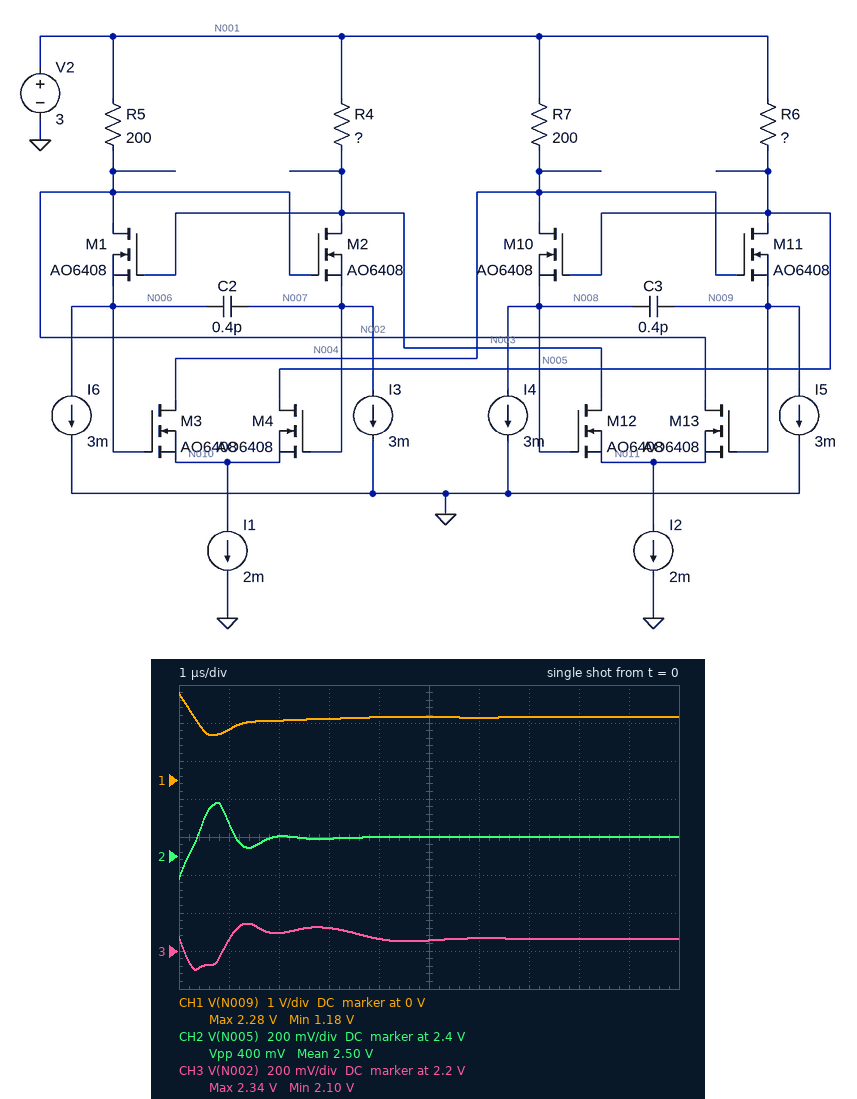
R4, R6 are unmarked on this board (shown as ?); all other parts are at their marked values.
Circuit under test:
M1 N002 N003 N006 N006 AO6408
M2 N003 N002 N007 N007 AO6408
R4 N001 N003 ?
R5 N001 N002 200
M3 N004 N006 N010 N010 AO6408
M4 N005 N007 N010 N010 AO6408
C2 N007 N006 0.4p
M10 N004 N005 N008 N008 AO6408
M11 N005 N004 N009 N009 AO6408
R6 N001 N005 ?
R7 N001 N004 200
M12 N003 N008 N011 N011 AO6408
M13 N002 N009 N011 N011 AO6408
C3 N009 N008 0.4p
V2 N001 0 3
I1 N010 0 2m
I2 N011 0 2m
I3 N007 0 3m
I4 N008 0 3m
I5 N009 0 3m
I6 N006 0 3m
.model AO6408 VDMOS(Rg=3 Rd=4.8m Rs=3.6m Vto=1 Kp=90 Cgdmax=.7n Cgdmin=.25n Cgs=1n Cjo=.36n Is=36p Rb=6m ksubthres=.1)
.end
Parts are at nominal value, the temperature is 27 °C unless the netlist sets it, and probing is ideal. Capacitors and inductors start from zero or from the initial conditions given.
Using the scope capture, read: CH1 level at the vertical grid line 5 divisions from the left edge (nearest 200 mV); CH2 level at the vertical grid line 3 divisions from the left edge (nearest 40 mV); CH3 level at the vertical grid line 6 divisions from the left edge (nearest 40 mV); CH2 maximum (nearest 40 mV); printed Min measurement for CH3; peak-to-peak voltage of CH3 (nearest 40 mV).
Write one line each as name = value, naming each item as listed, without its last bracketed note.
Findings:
CH1 level at the vertical grid line 5 divisions from the left edge = 1.6 V
CH2 level at the vertical grid line 3 divisions from the left edge = 2.48 V
CH3 level at the vertical grid line 6 divisions from the left edge = 2.28 V
CH2 maximum = 2.68 V
printed Min measurement for CH3 = 2.10 V
peak-to-peak voltage of CH3 = 240 mV
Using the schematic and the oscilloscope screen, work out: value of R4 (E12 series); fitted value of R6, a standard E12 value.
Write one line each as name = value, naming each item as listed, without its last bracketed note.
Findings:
value of R4 = 470 Ω
fitted value of R6, a standard E12 value = 100 Ω
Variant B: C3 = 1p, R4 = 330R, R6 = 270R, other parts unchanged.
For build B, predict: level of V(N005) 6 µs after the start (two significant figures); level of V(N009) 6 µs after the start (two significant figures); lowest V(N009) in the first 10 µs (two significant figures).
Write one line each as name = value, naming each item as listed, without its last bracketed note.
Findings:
level of V(N005) 6 µs after the start = 1.9 V
level of V(N009) 6 µs after the start = 1.4 V
lowest V(N009) in the first 10 µs = 1.3 V
